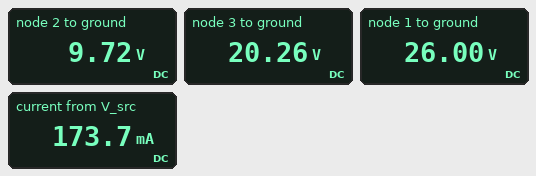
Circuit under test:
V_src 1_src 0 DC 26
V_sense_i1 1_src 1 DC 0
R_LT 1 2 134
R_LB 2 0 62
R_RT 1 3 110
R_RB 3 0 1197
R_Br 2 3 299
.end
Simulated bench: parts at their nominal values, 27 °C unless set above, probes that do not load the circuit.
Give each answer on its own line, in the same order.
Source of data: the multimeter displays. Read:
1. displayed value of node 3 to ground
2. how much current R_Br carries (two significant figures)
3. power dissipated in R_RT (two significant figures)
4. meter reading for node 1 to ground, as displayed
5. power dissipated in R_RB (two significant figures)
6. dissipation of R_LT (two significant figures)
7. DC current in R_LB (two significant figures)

20.26 V
35 mA
300 mW
26.00 V
340 mW
2.0 W
160 mA
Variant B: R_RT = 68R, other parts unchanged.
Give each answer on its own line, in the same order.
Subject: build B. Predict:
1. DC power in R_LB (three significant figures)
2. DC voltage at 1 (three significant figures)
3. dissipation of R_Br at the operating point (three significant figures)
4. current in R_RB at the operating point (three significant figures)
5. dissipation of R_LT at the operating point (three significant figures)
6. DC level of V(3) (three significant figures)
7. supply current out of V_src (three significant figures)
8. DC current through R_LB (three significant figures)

1.59 W
26.0 V
487 mW
18.4 mA
1.93 W
22.0 V
179 mA
160 mA
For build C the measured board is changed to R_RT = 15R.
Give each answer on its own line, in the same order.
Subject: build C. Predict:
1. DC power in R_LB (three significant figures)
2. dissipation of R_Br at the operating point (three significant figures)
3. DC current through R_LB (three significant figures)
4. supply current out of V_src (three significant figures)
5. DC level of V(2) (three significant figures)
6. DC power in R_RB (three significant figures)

1.71 W
718 mW
166 mA
187 mA
10.3 V
520 mW
